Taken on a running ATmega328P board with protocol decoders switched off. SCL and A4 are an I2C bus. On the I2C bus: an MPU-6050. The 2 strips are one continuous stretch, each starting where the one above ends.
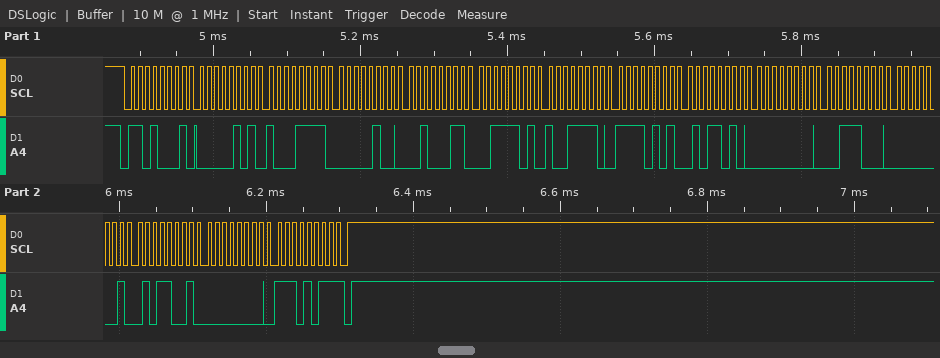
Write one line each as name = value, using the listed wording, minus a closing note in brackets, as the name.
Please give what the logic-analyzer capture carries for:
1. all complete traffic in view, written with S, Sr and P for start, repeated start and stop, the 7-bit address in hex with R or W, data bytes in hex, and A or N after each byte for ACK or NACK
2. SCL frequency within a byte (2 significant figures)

all complete traffic in view, written with S, Sr and P for start, repeated start and stop, the 7-bit address in hex with R or W, data bytes in hex, and A or N after each byte for ACK or NACK = S 68R A 05 A 8F A 04 A 23 A 3D A 9E A F5 A 5A A 00 A 38 A 01 A 59 A 00 A EB N P
SCL frequency within a byte = 100 kHz
